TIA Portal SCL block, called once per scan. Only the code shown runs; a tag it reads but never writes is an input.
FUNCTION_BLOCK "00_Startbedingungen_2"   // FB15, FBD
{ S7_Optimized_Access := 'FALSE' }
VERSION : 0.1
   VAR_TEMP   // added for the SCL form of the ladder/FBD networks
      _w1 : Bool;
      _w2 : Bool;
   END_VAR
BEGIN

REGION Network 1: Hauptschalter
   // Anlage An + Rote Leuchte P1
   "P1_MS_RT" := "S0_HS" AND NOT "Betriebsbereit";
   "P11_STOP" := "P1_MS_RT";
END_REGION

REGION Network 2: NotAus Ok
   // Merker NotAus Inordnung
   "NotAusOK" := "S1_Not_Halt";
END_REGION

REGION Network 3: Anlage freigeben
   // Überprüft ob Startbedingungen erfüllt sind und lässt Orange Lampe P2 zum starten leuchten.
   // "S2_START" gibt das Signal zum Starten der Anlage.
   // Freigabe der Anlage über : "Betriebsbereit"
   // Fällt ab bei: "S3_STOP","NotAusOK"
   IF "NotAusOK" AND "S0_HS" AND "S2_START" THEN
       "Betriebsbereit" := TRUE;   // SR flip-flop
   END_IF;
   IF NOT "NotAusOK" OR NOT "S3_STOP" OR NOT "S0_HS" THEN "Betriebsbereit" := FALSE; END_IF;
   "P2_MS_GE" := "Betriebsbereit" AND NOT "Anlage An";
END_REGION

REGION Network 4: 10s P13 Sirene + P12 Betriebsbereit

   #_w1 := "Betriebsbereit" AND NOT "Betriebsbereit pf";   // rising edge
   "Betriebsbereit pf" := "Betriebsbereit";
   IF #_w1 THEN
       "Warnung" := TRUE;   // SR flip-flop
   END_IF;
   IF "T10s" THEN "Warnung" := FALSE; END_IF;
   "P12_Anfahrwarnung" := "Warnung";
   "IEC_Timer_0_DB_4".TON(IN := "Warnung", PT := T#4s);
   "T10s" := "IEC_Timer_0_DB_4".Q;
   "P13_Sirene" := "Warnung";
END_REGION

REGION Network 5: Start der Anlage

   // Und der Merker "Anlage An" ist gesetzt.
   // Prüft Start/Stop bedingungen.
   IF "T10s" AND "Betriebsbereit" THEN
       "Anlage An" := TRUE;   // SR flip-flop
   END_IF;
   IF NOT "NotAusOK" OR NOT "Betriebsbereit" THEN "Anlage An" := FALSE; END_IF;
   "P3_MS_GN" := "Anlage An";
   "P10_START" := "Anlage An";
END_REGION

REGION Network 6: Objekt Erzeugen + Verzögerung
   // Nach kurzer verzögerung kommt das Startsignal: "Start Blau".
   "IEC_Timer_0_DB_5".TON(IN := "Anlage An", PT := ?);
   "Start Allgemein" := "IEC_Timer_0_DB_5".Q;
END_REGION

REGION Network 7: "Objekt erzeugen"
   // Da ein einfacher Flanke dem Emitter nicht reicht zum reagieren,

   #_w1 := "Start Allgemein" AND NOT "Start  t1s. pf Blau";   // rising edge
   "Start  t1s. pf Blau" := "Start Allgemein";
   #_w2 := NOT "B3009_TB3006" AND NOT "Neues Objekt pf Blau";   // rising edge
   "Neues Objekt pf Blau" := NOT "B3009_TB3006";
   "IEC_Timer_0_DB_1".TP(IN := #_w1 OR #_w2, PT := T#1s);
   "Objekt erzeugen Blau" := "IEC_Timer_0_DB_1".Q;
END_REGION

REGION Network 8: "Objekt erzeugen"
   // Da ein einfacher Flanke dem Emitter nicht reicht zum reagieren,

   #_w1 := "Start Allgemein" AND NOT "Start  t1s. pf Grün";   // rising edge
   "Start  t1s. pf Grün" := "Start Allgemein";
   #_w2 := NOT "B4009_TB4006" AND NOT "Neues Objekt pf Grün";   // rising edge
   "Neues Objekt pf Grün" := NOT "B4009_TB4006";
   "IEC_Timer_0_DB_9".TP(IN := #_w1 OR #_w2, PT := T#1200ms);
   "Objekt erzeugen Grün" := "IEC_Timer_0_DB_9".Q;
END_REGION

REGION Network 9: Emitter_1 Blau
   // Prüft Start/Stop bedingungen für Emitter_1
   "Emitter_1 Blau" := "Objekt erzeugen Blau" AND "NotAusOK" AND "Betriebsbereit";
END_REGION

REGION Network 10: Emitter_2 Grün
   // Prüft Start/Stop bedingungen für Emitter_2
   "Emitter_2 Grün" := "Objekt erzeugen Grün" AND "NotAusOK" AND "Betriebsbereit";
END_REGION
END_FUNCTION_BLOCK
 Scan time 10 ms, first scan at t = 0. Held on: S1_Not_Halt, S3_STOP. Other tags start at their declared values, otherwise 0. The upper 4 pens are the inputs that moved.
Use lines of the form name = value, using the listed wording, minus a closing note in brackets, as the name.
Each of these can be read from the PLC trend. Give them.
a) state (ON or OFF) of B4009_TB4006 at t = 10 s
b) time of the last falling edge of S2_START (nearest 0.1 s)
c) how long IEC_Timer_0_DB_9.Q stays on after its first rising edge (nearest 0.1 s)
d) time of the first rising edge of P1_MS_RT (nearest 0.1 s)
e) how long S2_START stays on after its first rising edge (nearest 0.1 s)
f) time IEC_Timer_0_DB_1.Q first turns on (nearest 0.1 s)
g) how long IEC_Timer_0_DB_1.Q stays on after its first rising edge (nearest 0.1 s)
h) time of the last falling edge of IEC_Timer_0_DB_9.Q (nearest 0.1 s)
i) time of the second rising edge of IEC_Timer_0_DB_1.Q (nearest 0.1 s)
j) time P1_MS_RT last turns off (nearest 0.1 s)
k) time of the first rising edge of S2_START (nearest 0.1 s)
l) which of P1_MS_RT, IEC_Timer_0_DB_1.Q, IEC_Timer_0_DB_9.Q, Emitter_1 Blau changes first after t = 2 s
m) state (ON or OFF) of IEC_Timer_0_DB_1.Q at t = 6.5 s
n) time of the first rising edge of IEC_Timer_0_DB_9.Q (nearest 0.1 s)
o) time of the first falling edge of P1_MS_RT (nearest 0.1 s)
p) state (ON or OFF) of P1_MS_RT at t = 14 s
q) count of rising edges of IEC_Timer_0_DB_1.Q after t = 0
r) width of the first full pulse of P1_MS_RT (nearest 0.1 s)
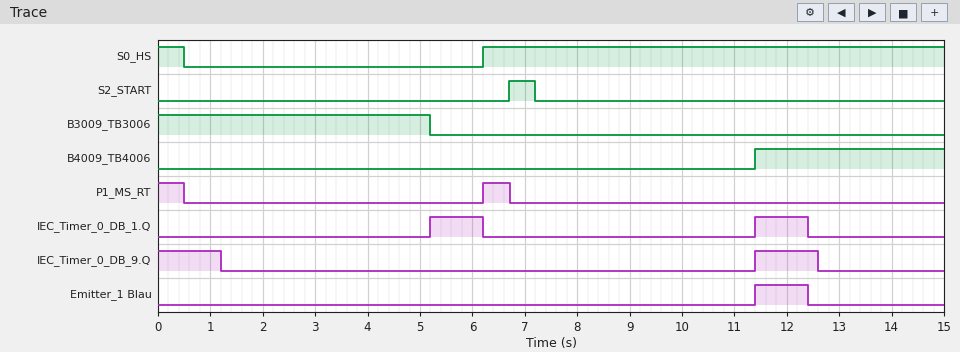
state (ON or OFF) of B4009_TB4006 at t = 10 s = OFF
time of the last falling edge of S2_START = 7.2 s
how long IEC_Timer_0_DB_9.Q stays on after its first rising edge = 1.2 s
time of the first rising edge of P1_MS_RT = 6.2 s
how long S2_START stays on after its first rising edge = 0.5 s
time IEC_Timer_0_DB_1.Q first turns on = 5.2 s
how long IEC_Timer_0_DB_1.Q stays on after its first rising edge = 1.0 s
time of the last falling edge of IEC_Timer_0_DB_9.Q = 12.6 s
time of the second rising edge of IEC_Timer_0_DB_1.Q = 11.4 s
time P1_MS_RT last turns off = 6.7 s
time of the first rising edge of S2_START = 6.7 s
which of P1_MS_RT, IEC_Timer_0_DB_1.Q, IEC_Timer_0_DB_9.Q, Emitter_1 Blau changes first after t = 2 s = IEC_Timer_0_DB_1.Q
state (ON or OFF) of IEC_Timer_0_DB_1.Q at t = 6.5 s = OFF
time of the first rising edge of IEC_Timer_0_DB_9.Q = 11.4 s
time of the first falling edge of P1_MS_RT = 0.5 s
state (ON or OFF) of P1_MS_RT at t = 14 s = OFF
count of rising edges of IEC_Timer_0_DB_1.Q after t = 0 = 2
width of the first full pulse of P1_MS_RT = 0.5 s
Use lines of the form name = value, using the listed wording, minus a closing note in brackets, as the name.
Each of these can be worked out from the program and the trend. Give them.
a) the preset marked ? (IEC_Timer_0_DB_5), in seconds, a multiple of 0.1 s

the preset marked ? (IEC_Timer_0_DB_5), in seconds, a multiple of 0.1 s = 0.7 s
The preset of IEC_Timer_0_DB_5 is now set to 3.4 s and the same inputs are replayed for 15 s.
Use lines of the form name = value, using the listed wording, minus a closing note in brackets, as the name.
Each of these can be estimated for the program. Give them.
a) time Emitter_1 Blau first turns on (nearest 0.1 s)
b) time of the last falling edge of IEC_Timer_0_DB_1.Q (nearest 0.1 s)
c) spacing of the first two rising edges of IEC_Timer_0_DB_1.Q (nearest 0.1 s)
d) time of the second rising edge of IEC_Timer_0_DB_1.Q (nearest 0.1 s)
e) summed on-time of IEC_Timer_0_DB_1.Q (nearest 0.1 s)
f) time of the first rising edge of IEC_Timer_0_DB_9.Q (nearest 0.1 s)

time Emitter_1 Blau first turns on = 14.1 s
time of the last falling edge of IEC_Timer_0_DB_1.Q = 6.2 s
spacing of the first two rising edges of IEC_Timer_0_DB_1.Q = 8.9 s
time of the second rising edge of IEC_Timer_0_DB_1.Q = 14.1 s
summed on-time of IEC_Timer_0_DB_1.Q = 1.9 s
time of the first rising edge of IEC_Timer_0_DB_9.Q = 14.1 s
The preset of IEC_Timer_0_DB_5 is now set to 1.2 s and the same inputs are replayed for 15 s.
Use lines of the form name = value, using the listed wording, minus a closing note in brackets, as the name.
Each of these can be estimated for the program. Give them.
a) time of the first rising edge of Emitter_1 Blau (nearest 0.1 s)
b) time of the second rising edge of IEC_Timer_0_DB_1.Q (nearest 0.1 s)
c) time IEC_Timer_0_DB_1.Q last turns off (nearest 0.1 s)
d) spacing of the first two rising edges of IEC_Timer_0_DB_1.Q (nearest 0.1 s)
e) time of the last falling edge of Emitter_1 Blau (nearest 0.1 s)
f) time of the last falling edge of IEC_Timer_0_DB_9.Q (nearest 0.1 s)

time of the first rising edge of Emitter_1 Blau = 11.9 s
time of the second rising edge of IEC_Timer_0_DB_1.Q = 11.9 s
time IEC_Timer_0_DB_1.Q last turns off = 12.9 s
spacing of the first two rising edges of IEC_Timer_0_DB_1.Q = 6.7 s
time of the last falling edge of Emitter_1 Blau = 12.9 s
time of the last falling edge of IEC_Timer_0_DB_9.Q = 13.1 s
